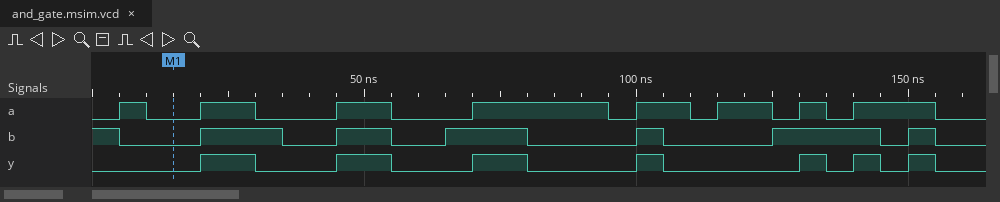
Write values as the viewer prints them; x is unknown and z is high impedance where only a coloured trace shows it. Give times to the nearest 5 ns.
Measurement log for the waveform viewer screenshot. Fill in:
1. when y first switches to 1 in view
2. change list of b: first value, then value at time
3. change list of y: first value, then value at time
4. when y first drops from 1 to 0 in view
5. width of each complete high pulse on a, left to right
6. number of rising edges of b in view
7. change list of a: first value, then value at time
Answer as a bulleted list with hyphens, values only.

- 20 ns
- 1, 0 at 5 ns, 1 at 20 ns, 0 at 35 ns, 1 at 45 ns, 0 at 55 ns, 1 at 65 ns, 0 at 80 ns, 1 at 100 ns, 0 at 105 ns, 1 at 125 ns, 0 at 145 ns, 1 at 150 ns, 0 at 155 ns
- 0, 1 at 20 ns, 0 at 30 ns, 1 at 45 ns, 0 at 55 ns, 1 at 70 ns, 0 at 80 ns, 1 at 100 ns, 0 at 105 ns, 1 at 130 ns, 0 at 135 ns, 1 at 140 ns, 0 at 145 ns, 1 at 150 ns, 0 at 155 ns
- 30 ns
- 5 ns, 10 ns, 10 ns, 25 ns, 10 ns, 10 ns, 5 ns, 15 ns
- 6
- 0, 1 at 5 ns, 0 at 10 ns, 1 at 20 ns, 0 at 30 ns, 1 at 45 ns, 0 at 55 ns, 1 at 70 ns, 0 at 95 ns, 1 at 100 ns, 0 at 110 ns, 1 at 115 ns, 0 at 125 ns, 1 at 130 ns, 0 at 135 ns, 1 at 140 ns, 0 at 155 ns
